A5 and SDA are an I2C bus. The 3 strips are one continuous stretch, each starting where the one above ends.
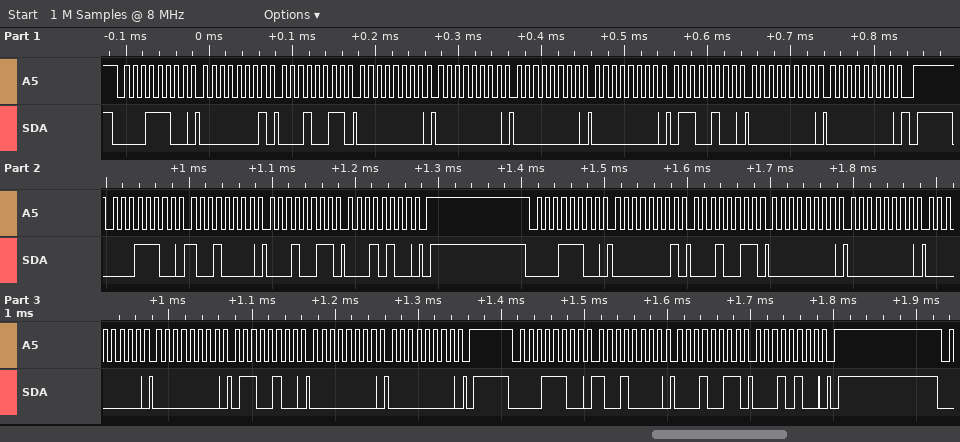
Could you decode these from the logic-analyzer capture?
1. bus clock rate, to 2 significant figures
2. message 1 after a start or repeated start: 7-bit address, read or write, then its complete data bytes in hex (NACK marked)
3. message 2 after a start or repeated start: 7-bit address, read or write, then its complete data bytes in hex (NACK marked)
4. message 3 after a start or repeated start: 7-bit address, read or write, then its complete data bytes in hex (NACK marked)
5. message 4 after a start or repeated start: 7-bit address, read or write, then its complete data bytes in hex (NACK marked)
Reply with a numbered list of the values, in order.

1. 100 kHz
2. 0x0E write: 01 13 00 00 00 00 64 00 00
3. 0x0E write: 90 13 14
4. 0x0E write: 01 13 00 00 00 00 64 00 00
5. 0x0E write: 90 13 14
